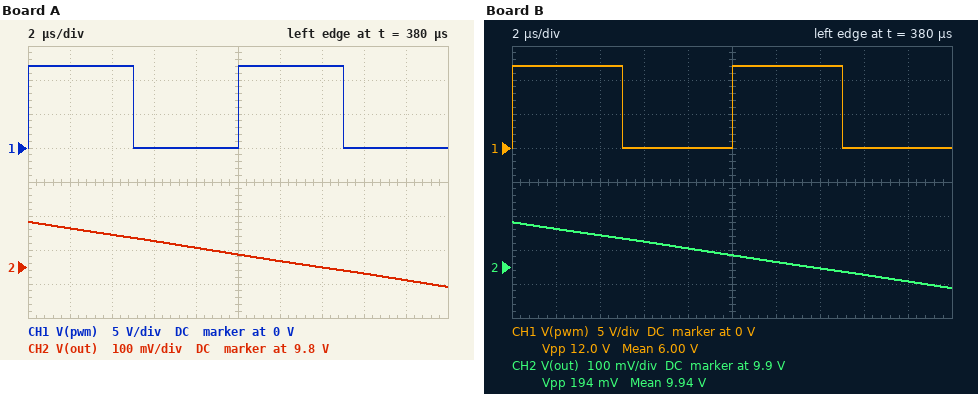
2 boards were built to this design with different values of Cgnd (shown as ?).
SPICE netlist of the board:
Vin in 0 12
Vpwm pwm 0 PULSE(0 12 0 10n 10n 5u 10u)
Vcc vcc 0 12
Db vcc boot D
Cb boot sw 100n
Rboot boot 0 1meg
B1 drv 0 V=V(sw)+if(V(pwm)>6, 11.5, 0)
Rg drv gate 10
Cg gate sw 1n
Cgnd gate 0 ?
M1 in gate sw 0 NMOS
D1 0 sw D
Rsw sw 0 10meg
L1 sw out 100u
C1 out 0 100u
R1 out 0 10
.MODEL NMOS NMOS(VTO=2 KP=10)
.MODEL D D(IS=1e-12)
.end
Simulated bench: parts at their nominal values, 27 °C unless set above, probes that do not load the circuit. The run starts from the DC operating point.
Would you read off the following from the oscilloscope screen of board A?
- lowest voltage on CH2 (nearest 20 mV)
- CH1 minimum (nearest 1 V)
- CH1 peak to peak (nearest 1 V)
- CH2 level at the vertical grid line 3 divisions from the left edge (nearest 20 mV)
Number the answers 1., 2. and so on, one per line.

1. 9.74 V
2. 0 V
3. 12 V
4. 9.88 V
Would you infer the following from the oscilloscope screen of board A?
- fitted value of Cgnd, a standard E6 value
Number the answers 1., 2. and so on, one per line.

1. 1.5 nF
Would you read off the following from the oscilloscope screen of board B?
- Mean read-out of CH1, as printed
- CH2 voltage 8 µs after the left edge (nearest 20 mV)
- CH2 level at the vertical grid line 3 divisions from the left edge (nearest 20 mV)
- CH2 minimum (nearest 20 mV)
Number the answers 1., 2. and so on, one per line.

1. 6.00 V
2. 9.96 V
3. 9.98 V
4. 9.84 V
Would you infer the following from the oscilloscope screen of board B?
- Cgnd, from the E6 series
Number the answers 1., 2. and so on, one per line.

1. 3.3 nF
